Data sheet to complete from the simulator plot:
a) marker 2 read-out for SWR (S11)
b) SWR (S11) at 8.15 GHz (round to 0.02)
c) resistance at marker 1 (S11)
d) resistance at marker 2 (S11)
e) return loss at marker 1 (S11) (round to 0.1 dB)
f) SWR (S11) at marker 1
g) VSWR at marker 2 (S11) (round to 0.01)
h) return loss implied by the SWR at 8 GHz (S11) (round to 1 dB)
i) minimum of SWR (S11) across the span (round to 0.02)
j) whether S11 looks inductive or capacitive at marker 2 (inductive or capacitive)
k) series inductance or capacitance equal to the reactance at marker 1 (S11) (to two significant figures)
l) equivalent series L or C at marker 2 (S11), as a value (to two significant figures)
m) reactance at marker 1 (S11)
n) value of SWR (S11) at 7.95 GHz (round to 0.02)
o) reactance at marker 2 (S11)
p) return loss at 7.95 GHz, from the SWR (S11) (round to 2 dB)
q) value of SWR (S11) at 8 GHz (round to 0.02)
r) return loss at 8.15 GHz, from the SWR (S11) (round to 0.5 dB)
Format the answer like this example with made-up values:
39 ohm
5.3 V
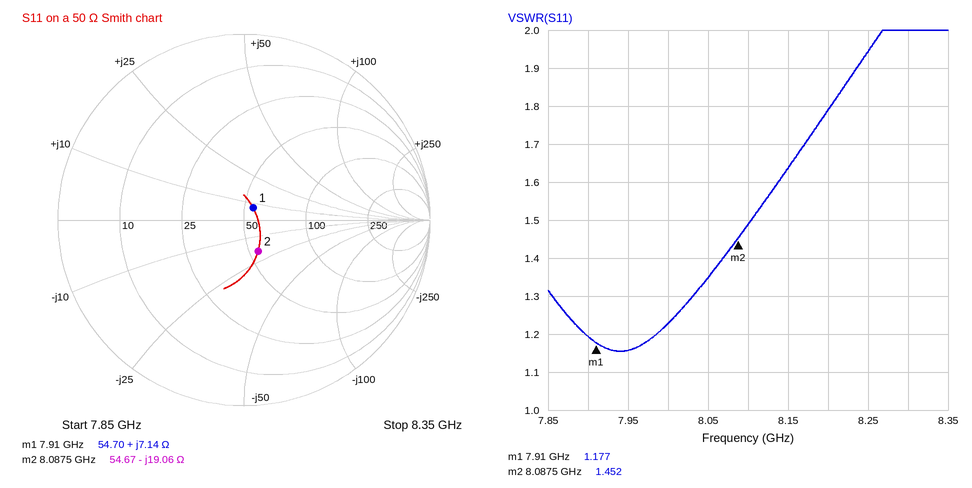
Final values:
1.452
1.64
54.70 Ω
54.67 Ω
21.8 dB
1.177
1.45
20 dB
1.16
capacitive
140 pH
1.0 pF
+7.14 Ω
1.16
-19.06 Ω
22 dB
1.22
12.5 dB
